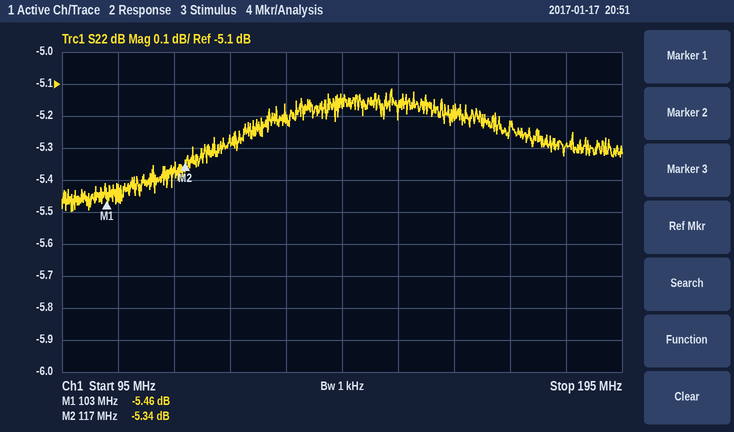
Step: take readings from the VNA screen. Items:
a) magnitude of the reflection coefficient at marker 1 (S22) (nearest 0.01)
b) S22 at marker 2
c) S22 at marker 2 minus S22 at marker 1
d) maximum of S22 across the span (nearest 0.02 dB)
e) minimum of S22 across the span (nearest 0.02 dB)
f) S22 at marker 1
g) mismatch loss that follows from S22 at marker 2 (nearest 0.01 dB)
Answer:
0.53
-5.34 dB
0.12 dB
-5.12 dB
-5.50 dB
-5.46 dB
1.50 dB
